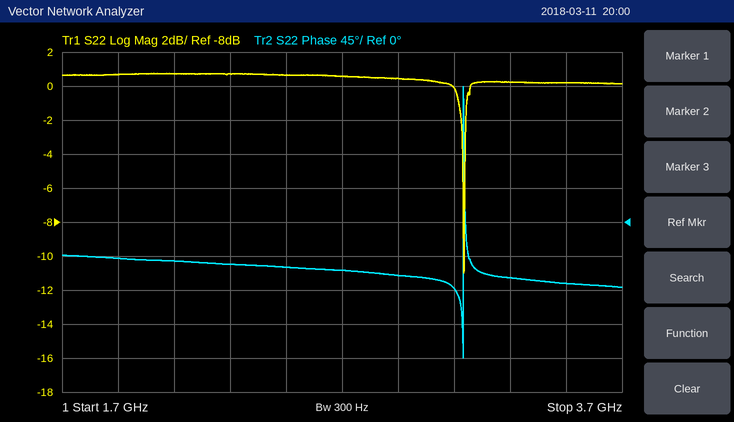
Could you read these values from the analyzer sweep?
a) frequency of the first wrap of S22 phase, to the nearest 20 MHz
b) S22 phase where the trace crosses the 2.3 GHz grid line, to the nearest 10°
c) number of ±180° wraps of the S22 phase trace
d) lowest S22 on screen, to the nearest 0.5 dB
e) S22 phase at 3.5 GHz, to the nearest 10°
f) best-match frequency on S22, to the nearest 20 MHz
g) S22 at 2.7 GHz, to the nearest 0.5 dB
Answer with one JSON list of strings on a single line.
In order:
["3.14 GHz", "-60°", "1", "-11.0 dB", "-80°", "3.14 GHz", "0.5 dB"]
